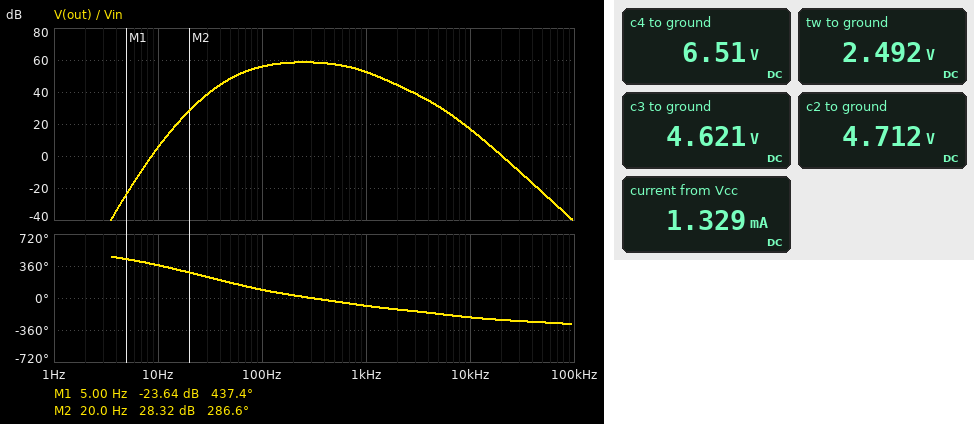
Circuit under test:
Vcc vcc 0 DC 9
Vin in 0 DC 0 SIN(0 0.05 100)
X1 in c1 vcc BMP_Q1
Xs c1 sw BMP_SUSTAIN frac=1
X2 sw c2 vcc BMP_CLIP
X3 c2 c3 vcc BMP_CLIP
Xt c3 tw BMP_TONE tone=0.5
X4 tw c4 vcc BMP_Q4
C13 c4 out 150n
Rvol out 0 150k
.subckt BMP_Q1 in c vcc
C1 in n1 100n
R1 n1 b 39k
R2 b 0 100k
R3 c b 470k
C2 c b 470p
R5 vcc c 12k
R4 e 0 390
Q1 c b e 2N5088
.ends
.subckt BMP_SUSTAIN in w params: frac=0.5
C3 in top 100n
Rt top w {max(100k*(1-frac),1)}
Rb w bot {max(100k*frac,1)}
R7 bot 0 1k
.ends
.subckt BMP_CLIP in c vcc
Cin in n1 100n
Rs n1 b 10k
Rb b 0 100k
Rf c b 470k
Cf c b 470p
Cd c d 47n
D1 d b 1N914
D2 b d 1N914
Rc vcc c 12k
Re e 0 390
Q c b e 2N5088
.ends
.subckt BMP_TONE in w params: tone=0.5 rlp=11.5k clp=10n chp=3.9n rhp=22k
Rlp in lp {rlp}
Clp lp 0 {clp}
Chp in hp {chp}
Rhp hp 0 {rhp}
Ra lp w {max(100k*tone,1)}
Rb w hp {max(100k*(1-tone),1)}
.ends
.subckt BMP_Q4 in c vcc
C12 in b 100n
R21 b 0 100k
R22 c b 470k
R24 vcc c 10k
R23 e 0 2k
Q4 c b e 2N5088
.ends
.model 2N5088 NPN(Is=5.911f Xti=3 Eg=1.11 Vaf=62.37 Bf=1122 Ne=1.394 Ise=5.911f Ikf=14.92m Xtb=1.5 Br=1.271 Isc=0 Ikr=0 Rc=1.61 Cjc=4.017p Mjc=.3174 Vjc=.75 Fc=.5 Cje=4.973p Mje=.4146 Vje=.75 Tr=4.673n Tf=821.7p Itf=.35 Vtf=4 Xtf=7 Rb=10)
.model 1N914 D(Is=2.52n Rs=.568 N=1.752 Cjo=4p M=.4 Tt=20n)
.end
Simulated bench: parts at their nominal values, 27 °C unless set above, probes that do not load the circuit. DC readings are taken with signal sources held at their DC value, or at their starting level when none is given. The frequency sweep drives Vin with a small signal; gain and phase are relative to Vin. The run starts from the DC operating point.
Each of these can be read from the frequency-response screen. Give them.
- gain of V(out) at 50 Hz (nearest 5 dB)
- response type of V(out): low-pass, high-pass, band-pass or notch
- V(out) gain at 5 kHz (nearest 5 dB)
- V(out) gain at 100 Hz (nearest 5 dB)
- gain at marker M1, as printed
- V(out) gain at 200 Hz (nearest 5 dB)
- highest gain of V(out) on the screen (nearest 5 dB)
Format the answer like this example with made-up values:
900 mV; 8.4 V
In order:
50 dB; band-pass; 30 dB; 55 dB; -23.64 dB; 60 dB; 60 dB
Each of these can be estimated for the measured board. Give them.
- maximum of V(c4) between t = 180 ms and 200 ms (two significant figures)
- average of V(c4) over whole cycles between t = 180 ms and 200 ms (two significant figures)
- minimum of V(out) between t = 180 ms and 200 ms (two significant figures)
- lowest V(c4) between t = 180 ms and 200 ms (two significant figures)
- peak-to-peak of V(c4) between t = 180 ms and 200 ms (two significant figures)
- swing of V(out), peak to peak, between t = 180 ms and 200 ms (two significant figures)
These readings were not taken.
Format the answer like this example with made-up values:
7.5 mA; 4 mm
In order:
7.7 V; 6.5 V; -1.2 V; 5.3 V; 2.4 V; 2.3 V
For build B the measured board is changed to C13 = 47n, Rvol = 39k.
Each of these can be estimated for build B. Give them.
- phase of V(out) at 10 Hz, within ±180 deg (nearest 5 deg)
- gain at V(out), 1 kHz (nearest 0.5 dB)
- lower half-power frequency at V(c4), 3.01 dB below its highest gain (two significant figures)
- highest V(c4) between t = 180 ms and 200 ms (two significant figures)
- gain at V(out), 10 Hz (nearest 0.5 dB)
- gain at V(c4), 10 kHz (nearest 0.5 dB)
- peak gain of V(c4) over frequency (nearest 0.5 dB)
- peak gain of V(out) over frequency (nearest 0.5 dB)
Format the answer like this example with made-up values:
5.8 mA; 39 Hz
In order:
55 deg; 51.5 dB; 87 Hz; 7.7 V; -11.5 dB; 15.5 dB; 57.5 dB; 57.0 dB
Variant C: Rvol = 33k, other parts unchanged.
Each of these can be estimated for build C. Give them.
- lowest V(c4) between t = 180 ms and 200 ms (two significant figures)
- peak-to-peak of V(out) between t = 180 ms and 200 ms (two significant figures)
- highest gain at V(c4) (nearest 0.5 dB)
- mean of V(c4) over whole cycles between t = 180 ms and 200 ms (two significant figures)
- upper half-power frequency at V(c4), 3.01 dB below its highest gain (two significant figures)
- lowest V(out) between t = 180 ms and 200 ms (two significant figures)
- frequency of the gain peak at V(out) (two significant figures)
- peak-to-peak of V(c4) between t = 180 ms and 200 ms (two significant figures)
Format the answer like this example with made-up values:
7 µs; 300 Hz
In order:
5.4 V; 1.8 V; 57.0 dB; 6.5 V; 690 Hz; -910 mV; 260 Hz; 2.1 V
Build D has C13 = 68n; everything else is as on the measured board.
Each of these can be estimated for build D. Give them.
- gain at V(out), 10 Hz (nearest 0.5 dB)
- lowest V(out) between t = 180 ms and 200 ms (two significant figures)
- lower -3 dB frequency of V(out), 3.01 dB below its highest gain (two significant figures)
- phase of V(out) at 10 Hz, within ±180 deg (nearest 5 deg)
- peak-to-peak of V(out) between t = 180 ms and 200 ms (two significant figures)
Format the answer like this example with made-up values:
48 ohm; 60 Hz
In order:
2.0 dB; -1.1 V; 96 Hz; 30 deg; 2.2 V
